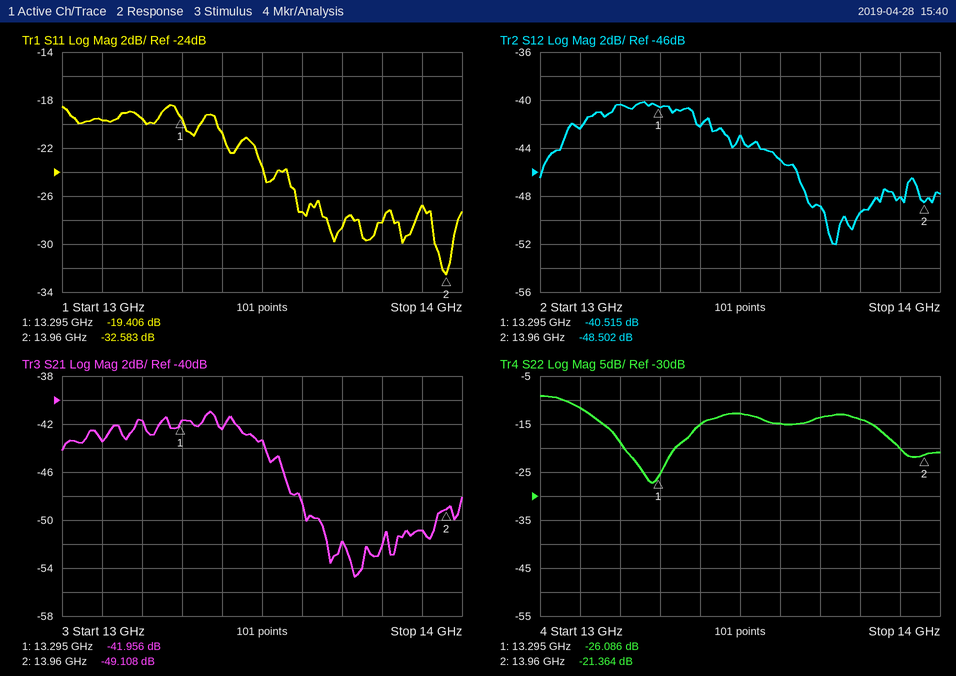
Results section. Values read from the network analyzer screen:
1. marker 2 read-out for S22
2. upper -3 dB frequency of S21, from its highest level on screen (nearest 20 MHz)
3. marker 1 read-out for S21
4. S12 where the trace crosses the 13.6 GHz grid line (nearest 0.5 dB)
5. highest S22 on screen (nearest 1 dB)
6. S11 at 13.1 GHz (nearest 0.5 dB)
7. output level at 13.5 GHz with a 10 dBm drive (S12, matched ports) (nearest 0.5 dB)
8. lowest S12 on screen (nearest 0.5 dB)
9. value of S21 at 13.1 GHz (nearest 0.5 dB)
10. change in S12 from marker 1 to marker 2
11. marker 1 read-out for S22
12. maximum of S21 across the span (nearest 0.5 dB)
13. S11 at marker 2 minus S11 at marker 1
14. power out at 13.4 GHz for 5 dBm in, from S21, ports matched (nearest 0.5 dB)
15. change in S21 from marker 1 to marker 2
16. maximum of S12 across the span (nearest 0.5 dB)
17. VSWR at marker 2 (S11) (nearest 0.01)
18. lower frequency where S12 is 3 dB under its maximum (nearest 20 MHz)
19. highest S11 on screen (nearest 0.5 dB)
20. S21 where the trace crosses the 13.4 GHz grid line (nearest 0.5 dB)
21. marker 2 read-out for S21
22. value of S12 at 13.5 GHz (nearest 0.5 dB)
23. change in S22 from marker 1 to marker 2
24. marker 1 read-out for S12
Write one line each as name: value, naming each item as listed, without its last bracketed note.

marker 2 read-out for S22: -21.364 dB
upper -3 dB frequency of S21, from its highest level on screen: 13.50 GHz
marker 1 read-out for S21: -41.956 dB
S12 where the trace crosses the 13.6 GHz grid line: -45.0 dB
highest S22 on screen: -9 dB
S11 at 13.1 GHz: -19.5 dB
output level at 13.5 GHz with a 10 dBm drive (S12, matched ports): -33.0 dBm
lowest S12 on screen: -52.0 dB
value of S21 at 13.1 GHz: -43.5 dB
change in S12 from marker 1 to marker 2: -7.987 dB
marker 1 read-out for S22: -26.086 dB
maximum of S21 across the span: -41.0 dB
S11 at marker 2 minus S11 at marker 1: -13.177 dB
power out at 13.4 GHz for 5 dBm in, from S21, ports matched: -37.5 dBm
change in S21 from marker 1 to marker 2: -7.152 dB
maximum of S12 across the span: -40.0 dB
VSWR at marker 2 (S11): 1.05
lower frequency where S12 is 3 dB under its maximum: 13.06 GHz
highest S11 on screen: -18.5 dB
S21 where the trace crosses the 13.4 GHz grid line: -42.5 dB
marker 2 read-out for S21: -49.108 dB
value of S12 at 13.5 GHz: -43.0 dB
change in S22 from marker 1 to marker 2: 4.722 dB
marker 1 read-out for S12: -40.515 dB
